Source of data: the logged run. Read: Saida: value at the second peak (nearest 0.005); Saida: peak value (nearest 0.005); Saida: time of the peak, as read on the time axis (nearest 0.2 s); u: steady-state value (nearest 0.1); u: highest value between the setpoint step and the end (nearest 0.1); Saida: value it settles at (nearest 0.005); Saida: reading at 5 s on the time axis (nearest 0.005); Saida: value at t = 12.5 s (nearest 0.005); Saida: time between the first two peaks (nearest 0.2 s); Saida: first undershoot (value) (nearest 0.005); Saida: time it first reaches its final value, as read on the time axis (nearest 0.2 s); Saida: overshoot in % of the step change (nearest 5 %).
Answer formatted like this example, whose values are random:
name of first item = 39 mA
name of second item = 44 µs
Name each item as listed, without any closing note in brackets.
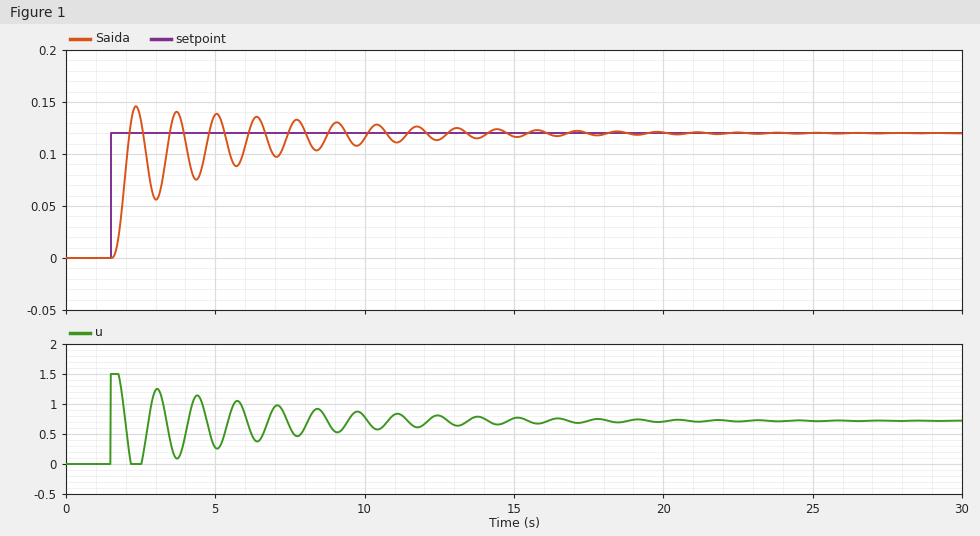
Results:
Saida: value at the second peak = 0.140
Saida: peak value = 0.145
Saida: time of the peak, as read on the time axis = 2.4 s
u: steady-state value = 0.7
u: highest value between the setpoint step and the end = 1.5
Saida: value it settles at = 0.120
Saida: reading at 5 s on the time axis = 0.140
Saida: value at t = 12.5 s = 0.115
Saida: time between the first two peaks = 1.4 s
Saida: first undershoot (value) = 0.055
Saida: time it first reaches its final value, as read on the time axis = 2.2 s
Saida: overshoot in % of the step change = 20 %
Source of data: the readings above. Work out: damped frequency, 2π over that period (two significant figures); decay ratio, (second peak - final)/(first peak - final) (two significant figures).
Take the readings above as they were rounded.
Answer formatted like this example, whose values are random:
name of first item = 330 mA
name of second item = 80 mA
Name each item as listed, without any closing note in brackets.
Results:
damped frequency, 2π over that period = 4.5 rad/s
decay ratio, (second peak - final)/(first peak - final) = 0.80
